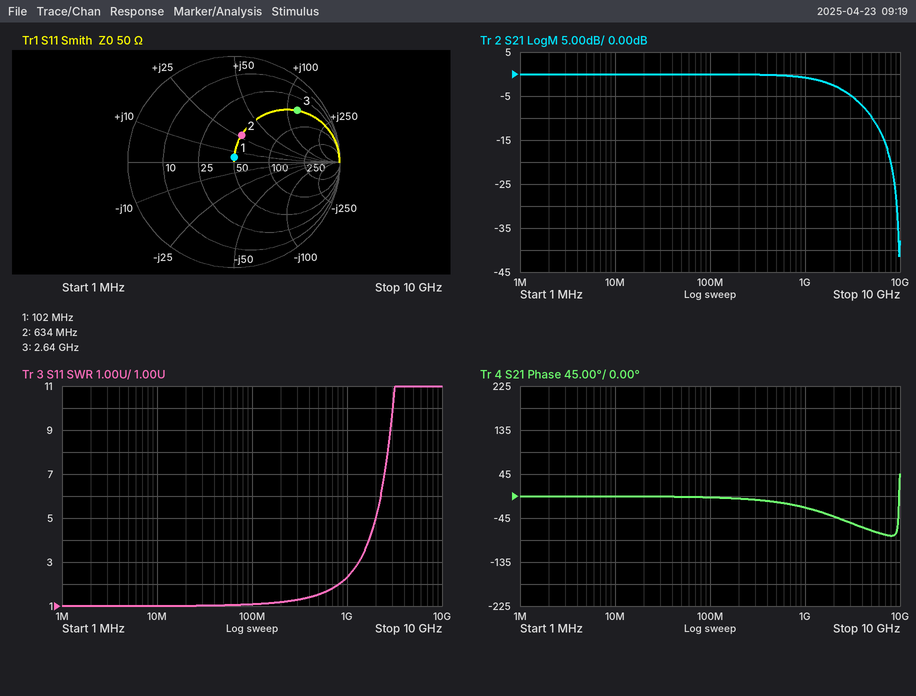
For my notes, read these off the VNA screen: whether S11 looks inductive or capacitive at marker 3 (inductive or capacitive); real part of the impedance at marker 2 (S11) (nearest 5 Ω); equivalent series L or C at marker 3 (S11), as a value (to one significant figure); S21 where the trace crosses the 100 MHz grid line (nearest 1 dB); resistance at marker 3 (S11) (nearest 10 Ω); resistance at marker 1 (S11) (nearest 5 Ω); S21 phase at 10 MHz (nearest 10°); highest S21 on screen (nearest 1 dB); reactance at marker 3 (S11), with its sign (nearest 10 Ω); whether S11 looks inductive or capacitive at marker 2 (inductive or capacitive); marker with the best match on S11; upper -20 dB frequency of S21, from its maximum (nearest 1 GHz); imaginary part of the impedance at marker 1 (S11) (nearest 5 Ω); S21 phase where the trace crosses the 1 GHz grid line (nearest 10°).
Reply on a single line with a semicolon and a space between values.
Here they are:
inductive; 50 Ω; 7 nH; 0 dB; 50 Ω; 50 Ω; 0°; 0 dB; +120 Ω; inductive; marker 1; 8 GHz; +5 Ω; -20°
